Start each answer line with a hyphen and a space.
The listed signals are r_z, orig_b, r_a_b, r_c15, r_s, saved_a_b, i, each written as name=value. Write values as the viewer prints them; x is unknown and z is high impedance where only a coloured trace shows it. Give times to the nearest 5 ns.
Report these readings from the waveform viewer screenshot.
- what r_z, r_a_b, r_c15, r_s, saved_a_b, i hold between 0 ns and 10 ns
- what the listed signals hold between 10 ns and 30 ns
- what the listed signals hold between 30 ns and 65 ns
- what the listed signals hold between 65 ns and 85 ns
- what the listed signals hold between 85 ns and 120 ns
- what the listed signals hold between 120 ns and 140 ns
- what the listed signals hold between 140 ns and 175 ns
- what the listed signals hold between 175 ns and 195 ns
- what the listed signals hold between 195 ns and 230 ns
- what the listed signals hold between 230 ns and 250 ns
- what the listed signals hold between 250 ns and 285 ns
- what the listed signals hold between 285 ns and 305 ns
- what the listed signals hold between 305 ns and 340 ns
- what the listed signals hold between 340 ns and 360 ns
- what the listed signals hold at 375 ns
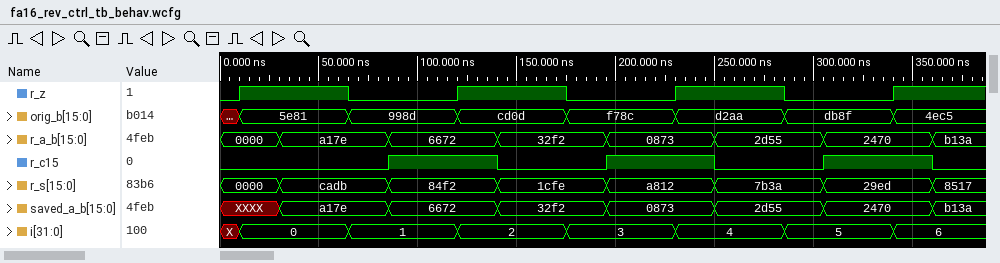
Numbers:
- r_z=0, r_a_b=0000, r_c15=0, r_s=0000, saved_a_b=XXXX, i=X
- r_z=1, orig_b=5e81, r_a_b=0000, r_c15=0, r_s=0000, saved_a_b=XXXX, i=0
- r_z=1, orig_b=5e81, r_a_b=a17e, r_c15=0, r_s=cadb, saved_a_b=a17e, i=0
- r_z=0, orig_b=998d, r_a_b=a17e, r_c15=0, r_s=cadb, saved_a_b=a17e, i=1
- r_z=0, orig_b=998d, r_a_b=6672, r_c15=1, r_s=84f2, saved_a_b=6672, i=1
- r_z=1, orig_b=cd0d, r_a_b=6672, r_c15=1, r_s=84f2, saved_a_b=6672, i=2
- r_z=1, orig_b=cd0d, r_a_b=32f2, r_c15=0, r_s=1cfe, saved_a_b=32f2, i=2
- r_z=0, orig_b=f78c, r_a_b=32f2, r_c15=0, r_s=1cfe, saved_a_b=32f2, i=3
- r_z=0, orig_b=f78c, r_a_b=0873, r_c15=1, r_s=a812, saved_a_b=0873, i=3
- r_z=1, orig_b=d2aa, r_a_b=0873, r_c15=1, r_s=a812, saved_a_b=0873, i=4
- r_z=1, orig_b=d2aa, r_a_b=2d55, r_c15=0, r_s=7b3a, saved_a_b=2d55, i=4
- r_z=0, orig_b=db8f, r_a_b=2d55, r_c15=0, r_s=7b3a, saved_a_b=2d55, i=5
- r_z=0, orig_b=db8f, r_a_b=2470, r_c15=1, r_s=29ed, saved_a_b=2470, i=5
- r_z=1, orig_b=4ec5, r_a_b=2470, r_c15=1, r_s=29ed, saved_a_b=2470, i=6
- r_z=1, orig_b=4ec5, r_a_b=b13a, r_c15=0, r_s=8517, saved_a_b=b13a, i=6
